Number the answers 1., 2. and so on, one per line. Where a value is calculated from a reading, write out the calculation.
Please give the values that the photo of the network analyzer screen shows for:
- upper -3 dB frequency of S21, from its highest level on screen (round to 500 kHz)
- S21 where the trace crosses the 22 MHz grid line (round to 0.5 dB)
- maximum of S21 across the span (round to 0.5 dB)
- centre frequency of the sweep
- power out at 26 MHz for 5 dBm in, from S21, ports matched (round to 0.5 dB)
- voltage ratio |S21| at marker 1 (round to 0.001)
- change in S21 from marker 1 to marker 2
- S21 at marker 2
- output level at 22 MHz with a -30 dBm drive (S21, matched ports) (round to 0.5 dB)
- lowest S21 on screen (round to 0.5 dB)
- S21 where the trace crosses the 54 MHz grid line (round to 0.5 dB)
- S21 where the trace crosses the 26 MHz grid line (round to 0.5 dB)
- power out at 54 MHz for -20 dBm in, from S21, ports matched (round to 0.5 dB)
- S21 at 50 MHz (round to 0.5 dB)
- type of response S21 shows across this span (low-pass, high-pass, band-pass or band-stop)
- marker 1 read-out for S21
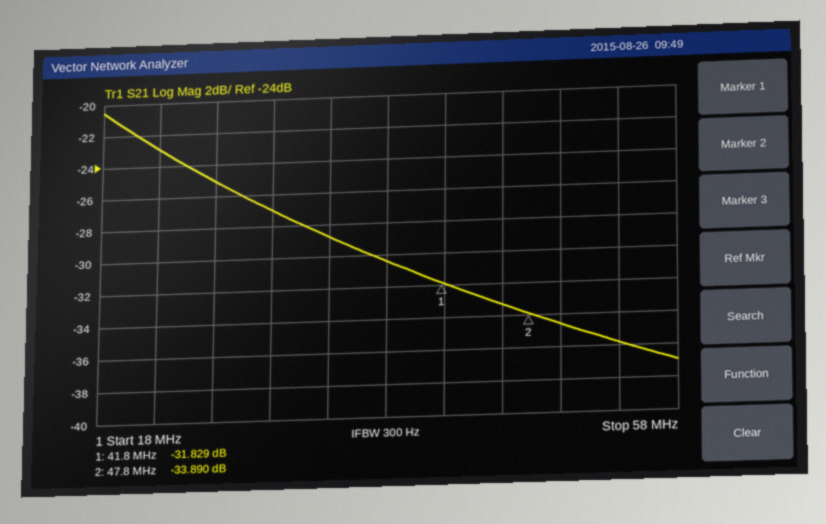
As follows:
1. 23.0 MHz
2. -23.0 dB
3. -20.5 dB
4. 38 MHz
5. 5 dBm + (-25.0 dB) = -20.0 dBm
6. 10^(-31.829/20) ≈ 0.026
7. -33.89 − (-31.829) = -2.061 dB
8. -33.890 dB
9. -30 dBm + (-23.0 dB) = -53.0 dBm
10. -37.0 dB
11. -36.0 dB
12. -25.0 dB
13. -20 dBm + (-36.0 dB) = -56.0 dBm
14. -34.5 dB
15. low-pass
16. -31.829 dB
